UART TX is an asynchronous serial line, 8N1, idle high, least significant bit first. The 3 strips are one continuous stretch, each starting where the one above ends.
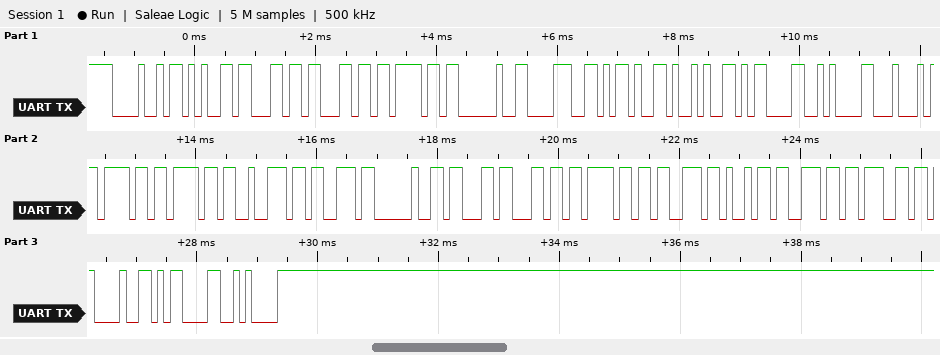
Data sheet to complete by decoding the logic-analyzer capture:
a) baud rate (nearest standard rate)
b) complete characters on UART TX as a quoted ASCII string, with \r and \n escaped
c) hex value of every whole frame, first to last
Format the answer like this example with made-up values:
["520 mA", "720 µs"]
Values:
["9600 baud", "\"Hello 8-)\\r\\nDoors closing!\\r\\n\"", "48 65 6C 6C 6F 20 38 2D 29 0D 0A 44 6F 6F 72 73 20 63 6C 6F 73 69 6E 67 21 0D 0A"]
